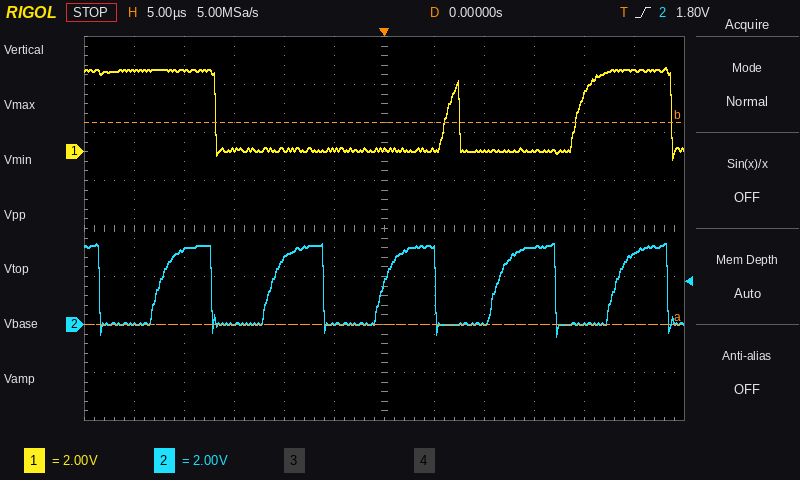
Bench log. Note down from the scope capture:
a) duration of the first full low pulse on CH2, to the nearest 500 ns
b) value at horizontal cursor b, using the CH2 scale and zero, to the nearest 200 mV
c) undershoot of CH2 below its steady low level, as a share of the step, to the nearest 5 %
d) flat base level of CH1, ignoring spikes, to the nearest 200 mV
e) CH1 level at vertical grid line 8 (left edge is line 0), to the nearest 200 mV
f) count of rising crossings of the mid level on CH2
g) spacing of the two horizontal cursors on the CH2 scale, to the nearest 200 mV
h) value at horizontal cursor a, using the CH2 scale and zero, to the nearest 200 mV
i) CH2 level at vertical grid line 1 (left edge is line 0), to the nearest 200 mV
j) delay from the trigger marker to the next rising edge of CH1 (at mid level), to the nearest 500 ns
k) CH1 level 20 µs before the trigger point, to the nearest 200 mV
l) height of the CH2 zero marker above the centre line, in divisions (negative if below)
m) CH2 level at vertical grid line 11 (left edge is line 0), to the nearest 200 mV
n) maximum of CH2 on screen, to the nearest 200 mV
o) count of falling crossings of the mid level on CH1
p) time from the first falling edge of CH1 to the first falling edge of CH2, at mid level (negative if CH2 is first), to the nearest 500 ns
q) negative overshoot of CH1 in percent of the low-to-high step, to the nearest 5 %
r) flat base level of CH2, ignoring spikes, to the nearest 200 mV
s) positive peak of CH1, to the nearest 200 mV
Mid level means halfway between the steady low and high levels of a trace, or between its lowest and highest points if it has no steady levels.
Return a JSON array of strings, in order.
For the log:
["6.0 µs", "8.4 V", "15 %", "0.0 V", "0.0 V", "5", "8.4 V", "0.0 V", "0.0 V", "6.5 µs", "3.4 V", "-2.0 div", "3.0 V", "3.4 V", "3", "-11.5 µs", "10 %", "0.0 V", "3.6 V"]
